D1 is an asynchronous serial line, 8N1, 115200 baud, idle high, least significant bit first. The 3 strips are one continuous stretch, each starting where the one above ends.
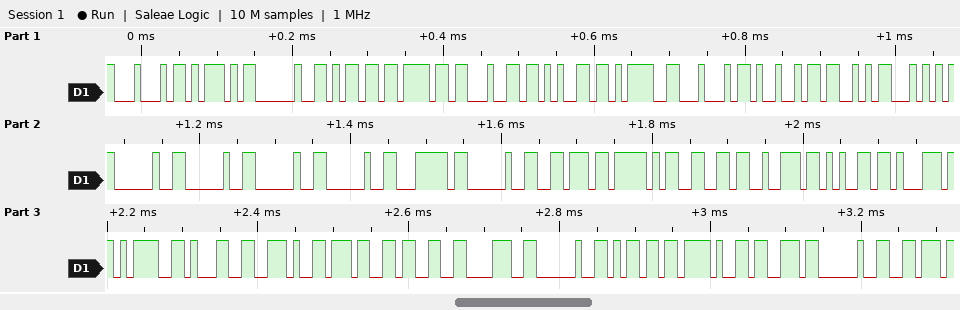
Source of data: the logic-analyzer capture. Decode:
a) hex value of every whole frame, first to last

0x44 0x5D 0x20 0x6D 0x6F 0x64 0x65 0x3D 0x44 0x49 0x53 0x54 0x20 0x20 0x20 0x20 0x7C 0x20 0x76 0x5F 0x66 0x72 0x65 0x71 0x3D 0x31 0x2E 0x37 0x33 0x38 0x20 0x6D 0x2F 0x73 0x20 0x76
